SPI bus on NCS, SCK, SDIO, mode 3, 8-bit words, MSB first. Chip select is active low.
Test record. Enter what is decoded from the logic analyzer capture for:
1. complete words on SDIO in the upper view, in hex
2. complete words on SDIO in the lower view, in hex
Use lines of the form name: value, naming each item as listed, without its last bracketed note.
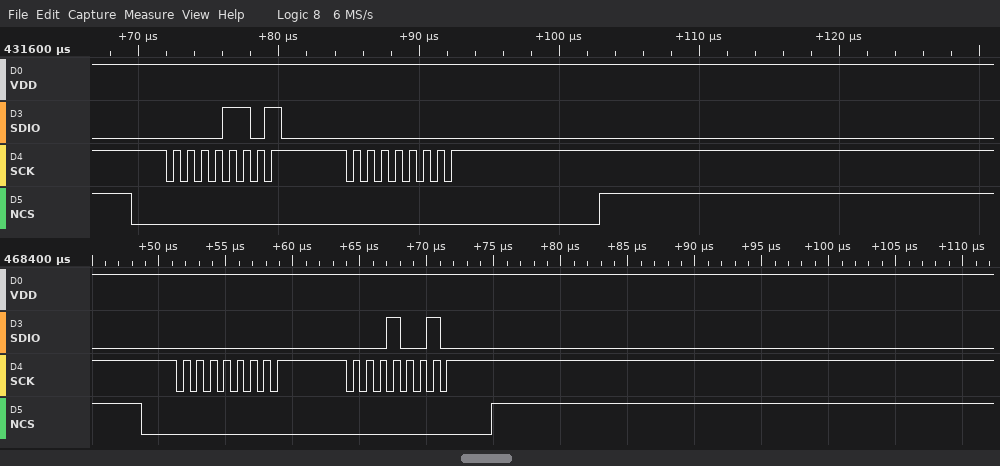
complete words on SDIO in the upper view, in hex: 0D, 00
complete words on SDIO in the lower view, in hex: 00, 12
